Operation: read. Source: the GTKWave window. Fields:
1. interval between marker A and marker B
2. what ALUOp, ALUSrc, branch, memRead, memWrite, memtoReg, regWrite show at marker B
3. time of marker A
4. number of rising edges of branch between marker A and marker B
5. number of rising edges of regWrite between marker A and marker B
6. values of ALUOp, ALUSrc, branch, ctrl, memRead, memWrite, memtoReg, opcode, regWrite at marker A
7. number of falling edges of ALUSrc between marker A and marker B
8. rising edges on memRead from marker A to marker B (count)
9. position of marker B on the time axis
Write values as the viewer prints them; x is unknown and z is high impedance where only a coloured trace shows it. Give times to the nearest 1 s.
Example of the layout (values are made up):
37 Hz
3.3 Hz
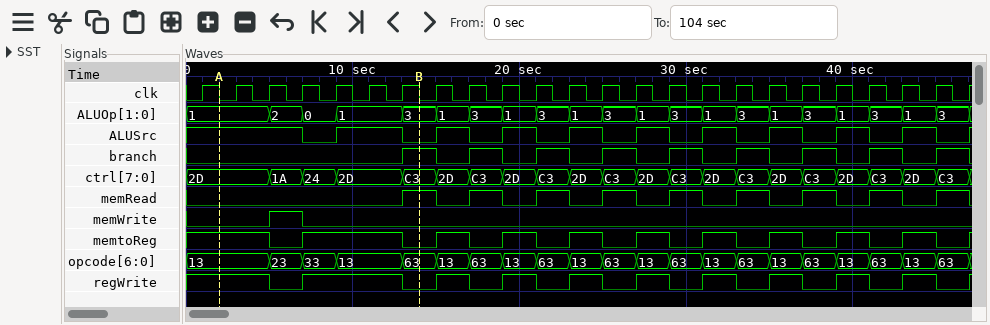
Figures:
12 s
ALUOp=3, ALUSrc=0, branch=1, memRead=1, memWrite=0, memtoReg=0, regWrite=0
2 s
1
1
ALUOp=1, ALUSrc=1, branch=0, ctrl=2D, memRead=0, memWrite=0, memtoReg=1, opcode=13, regWrite=1
2
1
14 s
